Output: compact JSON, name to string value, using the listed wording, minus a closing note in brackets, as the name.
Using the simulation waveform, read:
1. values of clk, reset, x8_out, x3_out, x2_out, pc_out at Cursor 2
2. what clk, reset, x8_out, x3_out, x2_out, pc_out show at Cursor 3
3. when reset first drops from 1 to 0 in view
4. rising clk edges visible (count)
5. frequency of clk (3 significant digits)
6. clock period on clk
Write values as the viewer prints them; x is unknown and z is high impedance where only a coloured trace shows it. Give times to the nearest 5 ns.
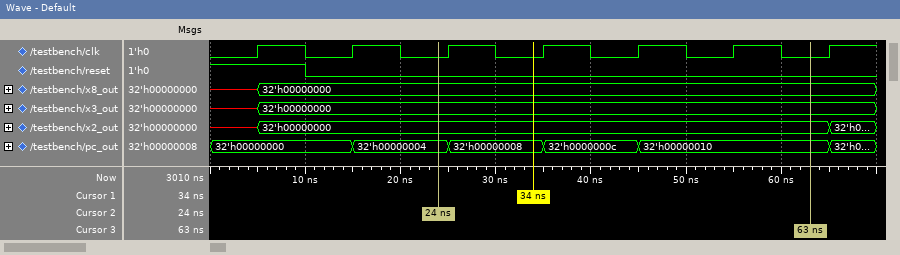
{"values of clk, reset, x8_out, x3_out, x2_out, pc_out at Cursor 2": "clk=0, reset=0, x8_out=32'h00000000, x3_out=32'h00000000, x2_out=32'h00000000, pc_out=32'h00000004", "what clk, reset, x8_out, x3_out, x2_out, pc_out show at Cursor 3": "clk=0, reset=0, x8_out=32'h00000000, x3_out=32'h00000000, x2_out=32'h00000000, pc_out=32'h00000010", "when reset first drops from 1 to 0 in view": "10 ns", "rising clk edges visible": "7", "frequency of clk": "100 MHz", "clock period on clk": "10 ns"}
